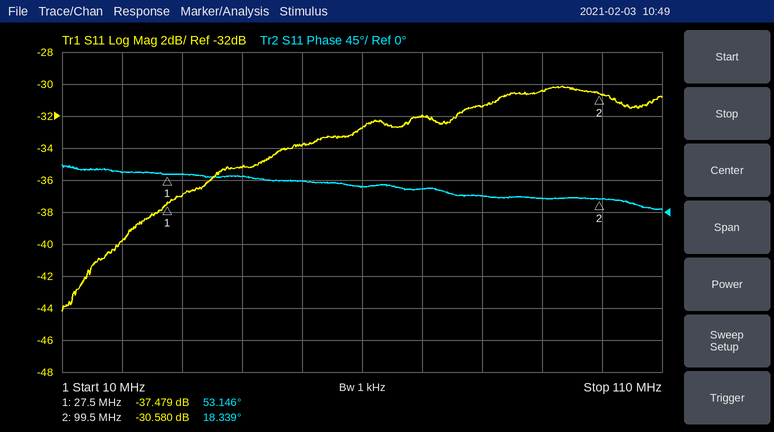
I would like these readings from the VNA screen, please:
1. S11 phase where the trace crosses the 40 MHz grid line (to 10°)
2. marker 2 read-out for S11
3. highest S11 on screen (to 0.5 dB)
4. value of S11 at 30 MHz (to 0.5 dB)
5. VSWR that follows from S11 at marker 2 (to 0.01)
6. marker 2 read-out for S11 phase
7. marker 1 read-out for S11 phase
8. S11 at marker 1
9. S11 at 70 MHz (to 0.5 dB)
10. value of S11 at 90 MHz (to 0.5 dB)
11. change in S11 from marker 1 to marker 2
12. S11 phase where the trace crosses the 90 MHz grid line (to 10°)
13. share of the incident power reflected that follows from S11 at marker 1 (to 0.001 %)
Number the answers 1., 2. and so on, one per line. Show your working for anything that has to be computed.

1. 50°
2. -30.580 dB
3. -30.0 dB
4. -37.0 dB
5. (1 + 0.0296)/(1 − 0.0296) ≈ 1.06
6. 18.339°
7. 53.146°
8. -37.479 dB
9. -32.0 dB
10. -30.5 dB
11. -30.58 − (-37.479) = 6.899 dB
12. 20°
13. 10^(-37.479/10) ≈ 0.018 %
